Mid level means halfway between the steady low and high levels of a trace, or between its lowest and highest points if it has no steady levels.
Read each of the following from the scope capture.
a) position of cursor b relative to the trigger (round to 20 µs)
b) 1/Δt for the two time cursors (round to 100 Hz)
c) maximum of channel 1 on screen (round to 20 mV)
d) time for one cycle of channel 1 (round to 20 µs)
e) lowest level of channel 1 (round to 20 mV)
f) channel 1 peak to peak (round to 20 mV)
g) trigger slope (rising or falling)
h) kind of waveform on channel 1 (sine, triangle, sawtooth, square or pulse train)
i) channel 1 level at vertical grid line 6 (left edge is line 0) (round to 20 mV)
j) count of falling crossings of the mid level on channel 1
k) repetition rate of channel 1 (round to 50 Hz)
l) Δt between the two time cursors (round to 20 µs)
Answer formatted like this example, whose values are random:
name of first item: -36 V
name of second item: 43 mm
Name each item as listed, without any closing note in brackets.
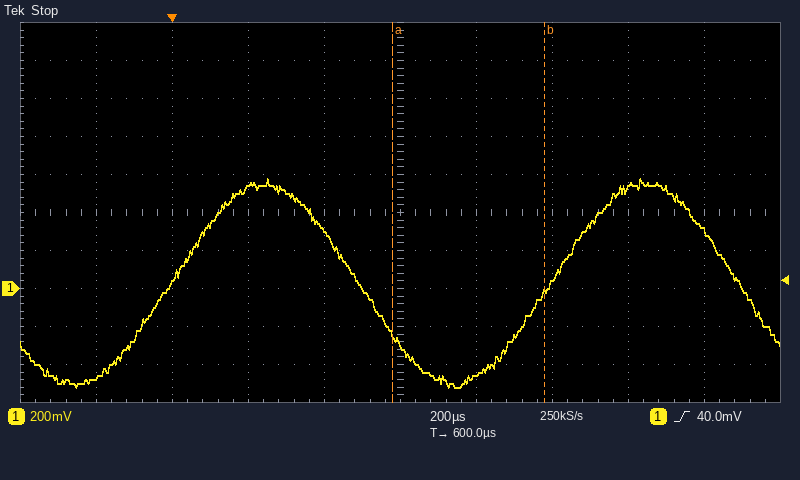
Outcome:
position of cursor b relative to the trigger: +980 µs
1/Δt for the two time cursors: 2.5 kHz
maximum of channel 1 on screen: 580 mV
time for one cycle of channel 1: 1.00 ms
lowest level of channel 1: -520 mV
channel 1 peak to peak: 1.10 V
trigger slope: rising
kind of waveform on channel 1: sine
channel 1 level at vertical grid line 6 (left edge is line 0): -460 mV
count of falling crossings of the mid level on channel 1: 2
repetition rate of channel 1: 1.00 kHz
Δt between the two time cursors: 400 µs
